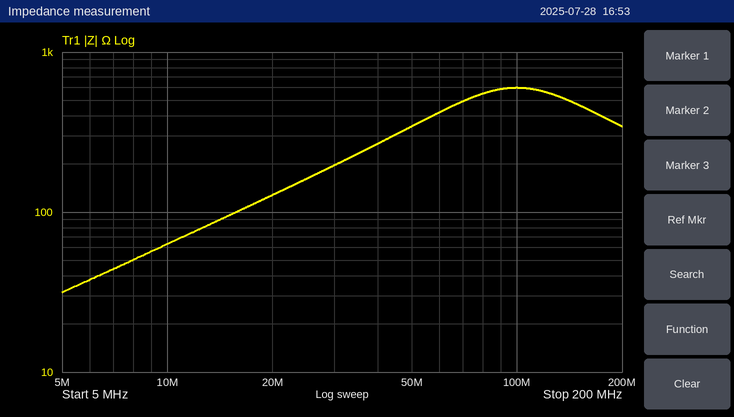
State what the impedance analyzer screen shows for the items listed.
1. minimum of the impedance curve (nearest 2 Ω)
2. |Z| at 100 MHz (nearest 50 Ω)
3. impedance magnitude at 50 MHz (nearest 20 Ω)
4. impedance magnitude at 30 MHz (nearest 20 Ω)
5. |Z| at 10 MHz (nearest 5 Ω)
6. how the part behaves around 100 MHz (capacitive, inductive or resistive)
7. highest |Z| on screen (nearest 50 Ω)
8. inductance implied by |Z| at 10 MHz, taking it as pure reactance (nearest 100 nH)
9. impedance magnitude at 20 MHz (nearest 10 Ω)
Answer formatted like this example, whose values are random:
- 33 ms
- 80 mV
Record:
- 32 Ω
- 600 Ω
- 340 Ω
- 200 Ω
- 65 Ω
- resistive
- 600 Ω
- 1.0 µH
- 130 Ω
